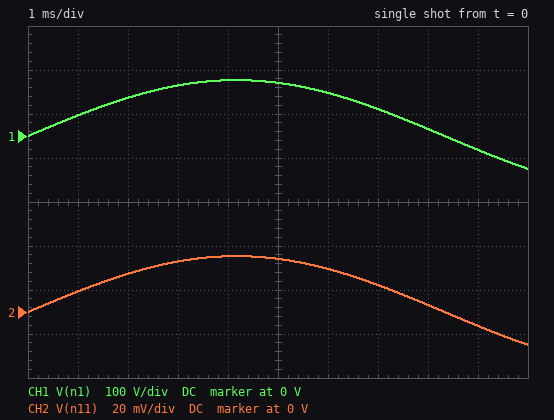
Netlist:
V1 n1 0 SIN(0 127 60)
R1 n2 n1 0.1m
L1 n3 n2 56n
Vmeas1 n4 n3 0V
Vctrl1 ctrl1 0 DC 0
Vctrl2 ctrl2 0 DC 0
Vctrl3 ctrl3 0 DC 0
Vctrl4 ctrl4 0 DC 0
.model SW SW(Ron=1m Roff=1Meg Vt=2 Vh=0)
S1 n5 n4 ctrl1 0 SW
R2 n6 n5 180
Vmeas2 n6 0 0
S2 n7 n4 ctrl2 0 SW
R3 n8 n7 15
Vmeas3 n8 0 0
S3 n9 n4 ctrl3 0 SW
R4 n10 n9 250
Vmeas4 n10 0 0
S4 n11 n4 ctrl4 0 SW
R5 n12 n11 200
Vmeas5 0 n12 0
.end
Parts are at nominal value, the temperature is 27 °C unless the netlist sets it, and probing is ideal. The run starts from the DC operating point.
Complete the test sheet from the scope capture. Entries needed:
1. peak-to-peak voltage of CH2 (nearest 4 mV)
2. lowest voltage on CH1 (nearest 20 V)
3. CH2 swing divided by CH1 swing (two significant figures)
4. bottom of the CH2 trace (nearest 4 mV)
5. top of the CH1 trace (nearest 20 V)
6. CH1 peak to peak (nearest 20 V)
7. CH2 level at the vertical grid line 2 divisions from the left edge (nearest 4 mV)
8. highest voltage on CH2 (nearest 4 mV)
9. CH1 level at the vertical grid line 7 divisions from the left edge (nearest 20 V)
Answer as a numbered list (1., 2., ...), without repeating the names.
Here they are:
1. 40 mV
2. -80 V
3. 0.00020
4. -16 mV
5. 120 V
6. 200 V
7. 16 mV
8. 24 mV
9. 60 V
